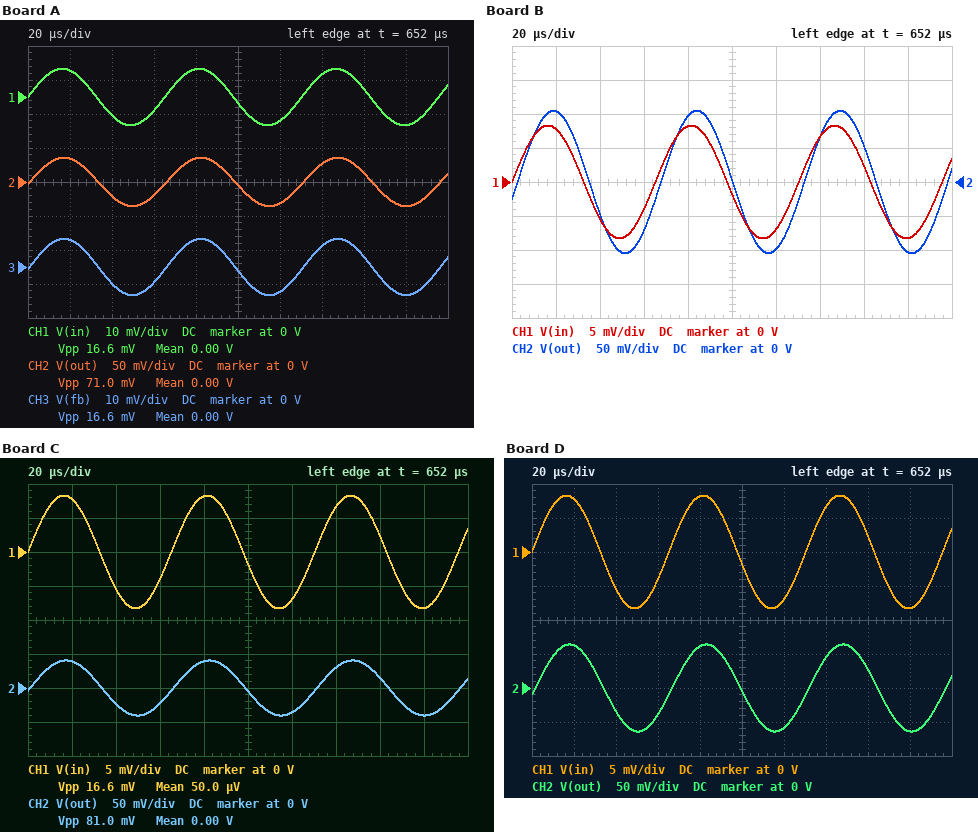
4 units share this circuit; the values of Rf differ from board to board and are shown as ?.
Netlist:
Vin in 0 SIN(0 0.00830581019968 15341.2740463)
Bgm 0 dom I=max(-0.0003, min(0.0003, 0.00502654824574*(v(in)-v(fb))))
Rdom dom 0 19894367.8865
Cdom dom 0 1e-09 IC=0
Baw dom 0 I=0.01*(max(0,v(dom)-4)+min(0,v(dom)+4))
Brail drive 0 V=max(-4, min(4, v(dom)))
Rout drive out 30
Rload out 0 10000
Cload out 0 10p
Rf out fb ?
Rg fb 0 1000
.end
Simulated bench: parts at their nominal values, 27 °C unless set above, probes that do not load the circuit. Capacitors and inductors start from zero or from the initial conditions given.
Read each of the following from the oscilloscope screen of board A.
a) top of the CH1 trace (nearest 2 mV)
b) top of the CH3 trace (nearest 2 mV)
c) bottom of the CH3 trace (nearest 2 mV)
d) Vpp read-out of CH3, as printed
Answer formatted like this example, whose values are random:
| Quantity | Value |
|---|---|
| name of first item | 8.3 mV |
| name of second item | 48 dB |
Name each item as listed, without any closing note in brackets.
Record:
| Quantity | Value |
|---|---|
| top of the CH1 trace | 8 mV |
| top of the CH3 trace | 8 mV |
| bottom of the CH3 trace | -8 mV |
| Vpp read-out of CH3, as printed | 16.6 mV |
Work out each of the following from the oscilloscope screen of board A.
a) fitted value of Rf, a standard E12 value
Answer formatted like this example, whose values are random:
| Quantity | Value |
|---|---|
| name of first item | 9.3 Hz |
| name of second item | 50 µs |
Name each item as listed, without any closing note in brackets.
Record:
| Quantity | Value |
|---|---|
| fitted value of Rf, a standard E12 value | 3.3 kΩ |
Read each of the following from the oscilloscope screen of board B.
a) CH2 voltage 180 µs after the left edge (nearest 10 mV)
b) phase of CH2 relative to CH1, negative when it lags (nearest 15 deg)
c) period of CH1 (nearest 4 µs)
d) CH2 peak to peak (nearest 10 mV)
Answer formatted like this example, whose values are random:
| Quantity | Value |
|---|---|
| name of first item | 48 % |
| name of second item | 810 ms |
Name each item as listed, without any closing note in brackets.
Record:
| Quantity | Value |
|---|---|
| CH2 voltage 180 µs after the left edge | -100 mV |
| phase of CH2 relative to CH1, negative when it lags | -15 deg |
| period of CH1 | 64 µs |
| CH2 peak to peak | 210 mV |
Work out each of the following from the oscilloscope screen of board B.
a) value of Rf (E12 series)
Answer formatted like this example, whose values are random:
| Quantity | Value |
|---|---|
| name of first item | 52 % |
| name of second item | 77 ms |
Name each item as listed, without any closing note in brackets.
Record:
| Quantity | Value |
|---|---|
| value of Rf | 12 kΩ |
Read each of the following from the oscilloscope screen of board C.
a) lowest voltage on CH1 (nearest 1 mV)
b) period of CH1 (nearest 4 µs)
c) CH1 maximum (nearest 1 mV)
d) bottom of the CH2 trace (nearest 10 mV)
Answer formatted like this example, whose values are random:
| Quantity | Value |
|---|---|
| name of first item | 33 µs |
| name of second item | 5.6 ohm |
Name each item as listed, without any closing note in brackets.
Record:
| Quantity | Value |
|---|---|
| lowest voltage on CH1 | -8 mV |
| period of CH1 | 64 µs |
| CH1 maximum | 8 mV |
| bottom of the CH2 trace | -40 mV |
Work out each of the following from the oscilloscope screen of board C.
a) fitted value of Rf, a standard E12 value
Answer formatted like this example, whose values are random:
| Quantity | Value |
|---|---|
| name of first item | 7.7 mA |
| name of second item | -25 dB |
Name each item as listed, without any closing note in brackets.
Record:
| Quantity | Value |
|---|---|
| fitted value of Rf, a standard E12 value | 3.9 kΩ |
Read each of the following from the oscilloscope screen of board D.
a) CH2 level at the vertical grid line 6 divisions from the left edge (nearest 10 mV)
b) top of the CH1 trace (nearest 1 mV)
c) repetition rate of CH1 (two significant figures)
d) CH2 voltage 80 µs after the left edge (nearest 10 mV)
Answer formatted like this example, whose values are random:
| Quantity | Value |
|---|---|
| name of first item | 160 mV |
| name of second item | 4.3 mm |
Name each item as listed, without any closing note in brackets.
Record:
| Quantity | Value |
|---|---|
| CH2 level at the vertical grid line 6 divisions from the left edge | -60 mV |
| top of the CH1 trace | 8 mV |
| repetition rate of CH1 | 15 kHz |
| CH2 voltage 80 µs after the left edge | 60 mV |
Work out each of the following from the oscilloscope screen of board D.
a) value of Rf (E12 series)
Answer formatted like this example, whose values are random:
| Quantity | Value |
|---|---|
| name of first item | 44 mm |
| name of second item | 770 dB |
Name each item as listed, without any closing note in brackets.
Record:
| Quantity | Value |
|---|---|
| value of Rf | 6.8 kΩ |
